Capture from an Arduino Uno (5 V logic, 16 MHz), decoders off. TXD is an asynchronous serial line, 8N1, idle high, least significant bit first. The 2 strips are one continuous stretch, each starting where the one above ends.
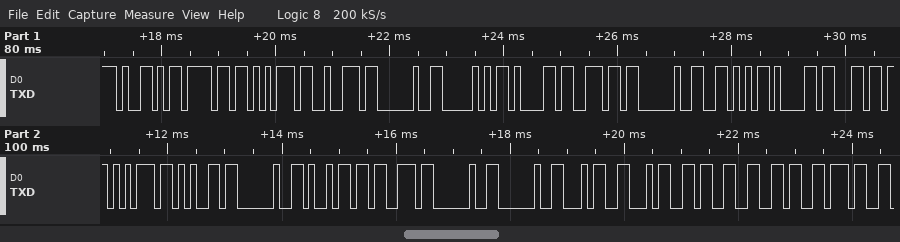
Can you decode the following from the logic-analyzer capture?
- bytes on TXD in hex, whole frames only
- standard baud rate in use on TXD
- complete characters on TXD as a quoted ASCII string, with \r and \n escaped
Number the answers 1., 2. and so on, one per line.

1. 59 6F 75 72 20 50 61 6E 20 56 61 6C 75 65 20 69 73 20 20 34 34 33 36 37
2. 9600 baud
3. "Your Pan Value is  44367"
